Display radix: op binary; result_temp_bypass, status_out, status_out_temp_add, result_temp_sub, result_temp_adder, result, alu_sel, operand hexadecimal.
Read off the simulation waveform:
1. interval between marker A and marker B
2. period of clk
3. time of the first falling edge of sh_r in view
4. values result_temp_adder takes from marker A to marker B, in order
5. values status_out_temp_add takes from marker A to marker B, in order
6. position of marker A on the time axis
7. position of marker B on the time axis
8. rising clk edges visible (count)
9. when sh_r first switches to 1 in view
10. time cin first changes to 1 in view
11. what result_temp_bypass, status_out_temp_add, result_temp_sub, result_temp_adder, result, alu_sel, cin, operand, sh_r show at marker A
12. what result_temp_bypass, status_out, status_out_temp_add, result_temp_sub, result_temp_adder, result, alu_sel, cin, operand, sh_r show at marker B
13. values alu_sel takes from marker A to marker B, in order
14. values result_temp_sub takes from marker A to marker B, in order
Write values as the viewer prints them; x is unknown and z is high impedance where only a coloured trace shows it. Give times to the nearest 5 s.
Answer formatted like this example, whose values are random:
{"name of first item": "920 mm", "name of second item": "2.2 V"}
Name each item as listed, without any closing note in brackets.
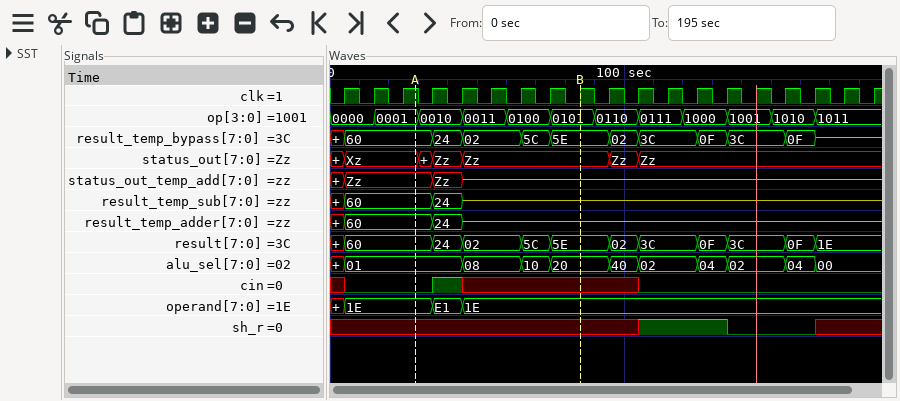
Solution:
{"interval between marker A and marker B": "55 s", "period of clk": "10 s", "time of the first falling edge of sh_r in view": "135 s", "values result_temp_adder takes from marker A to marker B, in order": "60, 24, z", "values status_out_temp_add takes from marker A to marker B, in order": "Zz, Zz, z", "position of marker A on the time axis": "30 s", "position of marker B on the time axis": "85 s", "rising clk edges visible": "19", "when sh_r first switches to 1 in view": "105 s", "time cin first changes to 1 in view": "35 s", "what result_temp_bypass, status_out_temp_add, result_temp_sub, result_temp_adder, result, alu_sel, cin, operand, sh_r show at marker A": "result_temp_bypass=60, status_out_temp_add=Zz, result_temp_sub=60, result_temp_adder=60, result=60, alu_sel=01, cin=0, operand=1E, sh_r=x", "what result_temp_bypass, status_out, status_out_temp_add, result_temp_sub, result_temp_adder, result, alu_sel, cin, operand, sh_r show at marker B": "result_temp_bypass=5E, status_out=Zz, status_out_temp_add=z, result_temp_sub=z, result_temp_adder=z, result=5E, alu_sel=20, cin=x, operand=1E, sh_r=x", "values alu_sel takes from marker A to marker B, in order": "01, 08, 10, 20", "values result_temp_sub takes from marker A to marker B, in order": "60, 24, z"}
